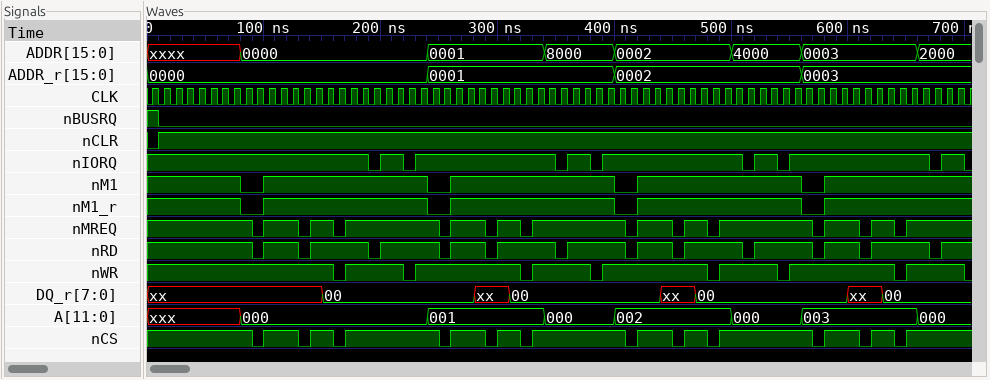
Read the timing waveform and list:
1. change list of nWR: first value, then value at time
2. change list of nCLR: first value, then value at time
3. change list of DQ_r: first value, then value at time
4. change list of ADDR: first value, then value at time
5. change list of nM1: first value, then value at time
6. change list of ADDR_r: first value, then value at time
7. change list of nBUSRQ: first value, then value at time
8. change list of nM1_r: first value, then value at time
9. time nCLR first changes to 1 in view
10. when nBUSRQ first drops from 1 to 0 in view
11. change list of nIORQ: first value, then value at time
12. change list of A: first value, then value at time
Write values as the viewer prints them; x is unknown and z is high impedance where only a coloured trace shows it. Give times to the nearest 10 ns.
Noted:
1, 0 at 160 ns, 1 at 170 ns, 0 at 220 ns, 1 at 230 ns, 0 at 320 ns, 1 at 330 ns, 0 at 380 ns, 1 at 390 ns, 0 at 480 ns, 1 at 490 ns, 0 at 540 ns, 1 at 550 ns, 0 at 640 ns, 1 at 650 ns, 0 at 700 ns
0, 1 at 10 ns
xx, 00 at 150 ns, xx at 280 ns, 00 at 310 ns, xx at 440 ns, 00 at 470 ns, xx at 600 ns, 00 at 630 ns
xxxx, 0000 at 80 ns, 0001 at 240 ns, 8000 at 340 ns, 0002 at 400 ns, 4000 at 500 ns, 0003 at 560 ns, 2000 at 660 ns
1, 0 at 80 ns, 1 at 100 ns, 0 at 240 ns, 1 at 260 ns, 0 at 400 ns, 1 at 420 ns, 0 at 560 ns, 1 at 580 ns
0000, 0001 at 240 ns, 0002 at 400 ns, 0003 at 560 ns
1, 0 at 10 ns
1, 0 at 80 ns, 1 at 100 ns, 0 at 240 ns, 1 at 260 ns, 0 at 400 ns, 1 at 420 ns, 0 at 560 ns, 1 at 580 ns
10 ns
10 ns
1, 0 at 190 ns, 1 at 200 ns, 0 at 220 ns, 1 at 230 ns, 0 at 350 ns, 1 at 360 ns, 0 at 380 ns, 1 at 390 ns, 0 at 510 ns, 1 at 520 ns, 0 at 540 ns, 1 at 550 ns, 0 at 670 ns, 1 at 680 ns, 0 at 700 ns
xxx, 000 at 80 ns, 001 at 240 ns, 000 at 340 ns, 002 at 400 ns, 000 at 500 ns, 003 at 560 ns, 000 at 660 ns
